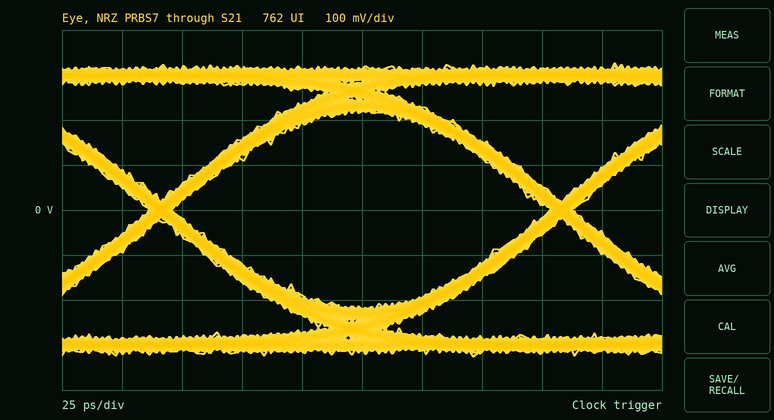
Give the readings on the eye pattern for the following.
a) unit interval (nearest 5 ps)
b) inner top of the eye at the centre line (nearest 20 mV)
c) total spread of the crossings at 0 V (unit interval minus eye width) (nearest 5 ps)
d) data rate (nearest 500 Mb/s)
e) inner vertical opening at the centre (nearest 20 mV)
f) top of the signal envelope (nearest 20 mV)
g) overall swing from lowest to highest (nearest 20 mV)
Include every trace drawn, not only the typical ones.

165 ps
220 mV
10 ps
6.0 Gb/s
440 mV
320 mV
660 mV
